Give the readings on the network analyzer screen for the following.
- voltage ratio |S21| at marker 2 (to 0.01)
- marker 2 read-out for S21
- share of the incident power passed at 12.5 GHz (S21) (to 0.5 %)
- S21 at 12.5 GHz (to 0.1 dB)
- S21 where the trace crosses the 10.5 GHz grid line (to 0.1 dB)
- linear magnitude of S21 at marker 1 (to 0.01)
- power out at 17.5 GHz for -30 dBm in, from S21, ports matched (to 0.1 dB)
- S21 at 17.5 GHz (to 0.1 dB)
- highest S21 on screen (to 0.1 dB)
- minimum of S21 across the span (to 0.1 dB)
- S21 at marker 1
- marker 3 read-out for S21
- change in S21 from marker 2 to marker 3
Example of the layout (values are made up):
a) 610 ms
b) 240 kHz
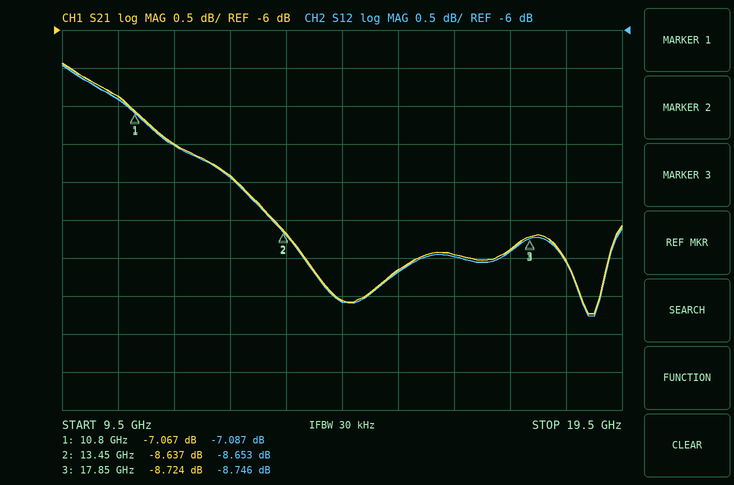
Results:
a) 0.37
b) -8.637 dB
c) 16.0 %
d) -7.9 dB
e) -6.9 dB
f) 0.44
g) -38.9 dBm
h) -8.9 dB
i) -6.4 dB
j) -9.7 dB
k) -7.067 dB
l) -8.724 dB
m) -0.087 dB
